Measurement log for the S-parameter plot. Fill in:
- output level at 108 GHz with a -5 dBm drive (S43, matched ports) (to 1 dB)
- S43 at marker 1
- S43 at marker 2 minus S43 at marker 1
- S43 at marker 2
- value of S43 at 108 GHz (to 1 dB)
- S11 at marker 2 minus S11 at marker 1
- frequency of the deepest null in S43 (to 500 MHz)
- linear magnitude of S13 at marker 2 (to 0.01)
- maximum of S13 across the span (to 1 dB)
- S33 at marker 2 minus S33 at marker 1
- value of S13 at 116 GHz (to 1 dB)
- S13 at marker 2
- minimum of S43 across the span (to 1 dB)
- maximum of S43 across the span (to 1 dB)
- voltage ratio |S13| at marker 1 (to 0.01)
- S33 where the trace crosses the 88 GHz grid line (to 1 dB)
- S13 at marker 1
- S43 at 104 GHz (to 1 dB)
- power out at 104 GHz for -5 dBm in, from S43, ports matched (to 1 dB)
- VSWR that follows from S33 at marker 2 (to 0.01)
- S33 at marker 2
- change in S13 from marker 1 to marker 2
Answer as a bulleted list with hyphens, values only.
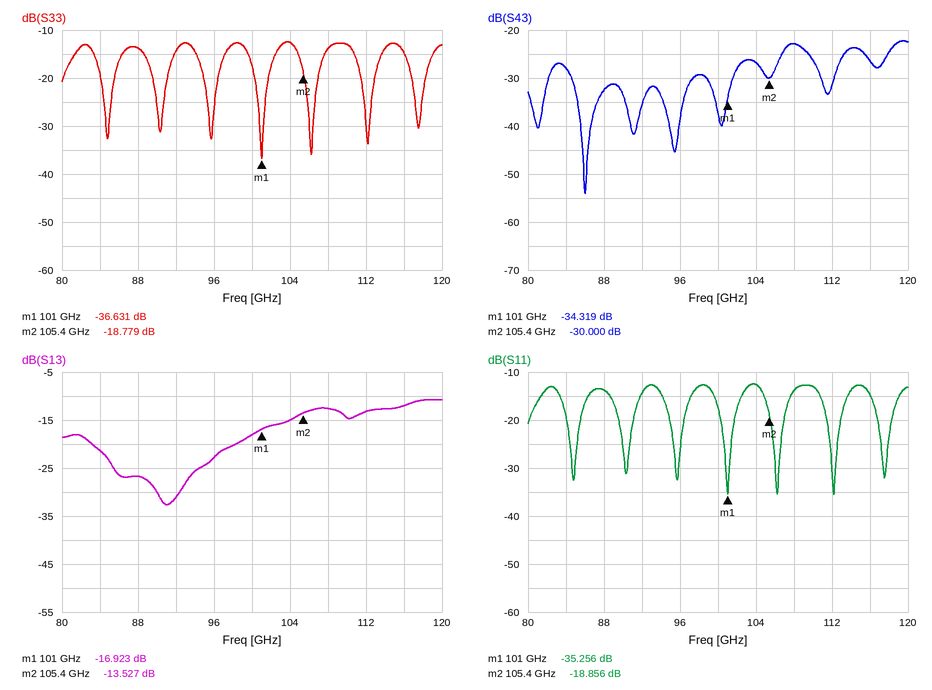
- -28 dBm
- -34.319 dB
- 4.319 dB
- -30.000 dB
- -23 dB
- 16.400 dB
- 86.0 GHz
- 0.21
- -11 dB
- 17.852 dB
- -12 dB
- -13.527 dB
- -54 dB
- -22 dB
- 0.14
- -14 dB
- -16.923 dB
- -27 dB
- -32 dBm
- 1.26
- -18.779 dB
- 3.396 dB
